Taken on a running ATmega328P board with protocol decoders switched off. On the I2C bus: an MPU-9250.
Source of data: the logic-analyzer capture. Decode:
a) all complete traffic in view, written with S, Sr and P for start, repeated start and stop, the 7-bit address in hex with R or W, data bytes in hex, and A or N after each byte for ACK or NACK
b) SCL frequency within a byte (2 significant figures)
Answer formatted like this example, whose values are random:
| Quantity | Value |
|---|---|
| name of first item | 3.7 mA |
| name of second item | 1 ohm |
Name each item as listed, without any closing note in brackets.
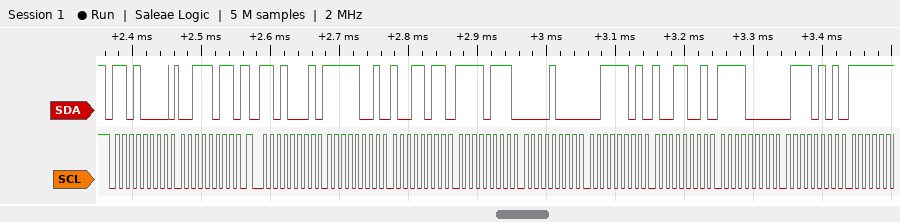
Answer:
| Quantity | Value |
|---|---|
| all complete traffic in view, written with S, Sr and P for start, repeated start and stop, the 7-bit address in hex with R or W, data bytes in hex, and A or N after each byte for ACK or NACK | S 68W A 3B A Sr 68R A F9 A 9B A F7 A 08 A 3D A 99 A F0 A 75 A |
| SCL frequency within a byte | 100 kHz |
